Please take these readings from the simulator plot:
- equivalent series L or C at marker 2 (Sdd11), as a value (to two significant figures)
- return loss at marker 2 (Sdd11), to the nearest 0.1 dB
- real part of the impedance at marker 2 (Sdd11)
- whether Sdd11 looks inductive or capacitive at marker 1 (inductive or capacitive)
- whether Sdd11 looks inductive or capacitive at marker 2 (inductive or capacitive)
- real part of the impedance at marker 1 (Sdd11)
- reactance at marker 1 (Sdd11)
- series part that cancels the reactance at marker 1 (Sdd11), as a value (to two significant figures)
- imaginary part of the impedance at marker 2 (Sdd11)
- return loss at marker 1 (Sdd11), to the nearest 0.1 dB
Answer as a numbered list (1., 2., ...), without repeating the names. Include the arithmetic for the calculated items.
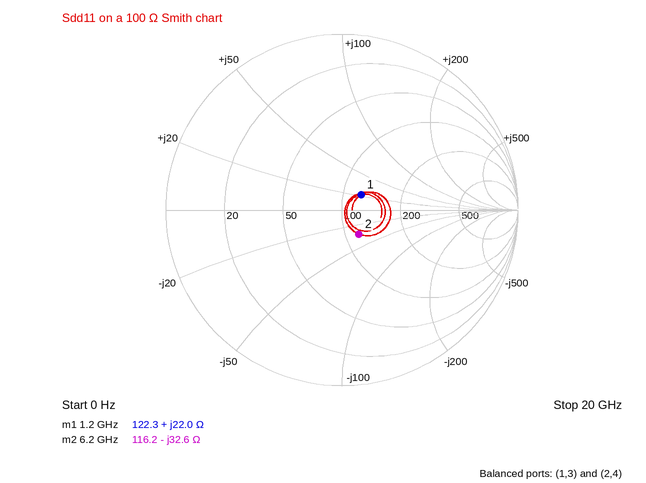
1. C = 1/(2π × 6.2 GHz × 32.6 Ω) ≈ 787 fF, so 790 fF to two significant figures
2. 15.6 dB
3. 116.2 Ω
4. inductive
5. capacitive
6. 122.3 Ω
7. +22.0 Ω
8. C = 1/(2π × 1.2 GHz × 22 Ω) ≈ 6.0 pF
9. -32.6 Ω
10. 17.1 dB
